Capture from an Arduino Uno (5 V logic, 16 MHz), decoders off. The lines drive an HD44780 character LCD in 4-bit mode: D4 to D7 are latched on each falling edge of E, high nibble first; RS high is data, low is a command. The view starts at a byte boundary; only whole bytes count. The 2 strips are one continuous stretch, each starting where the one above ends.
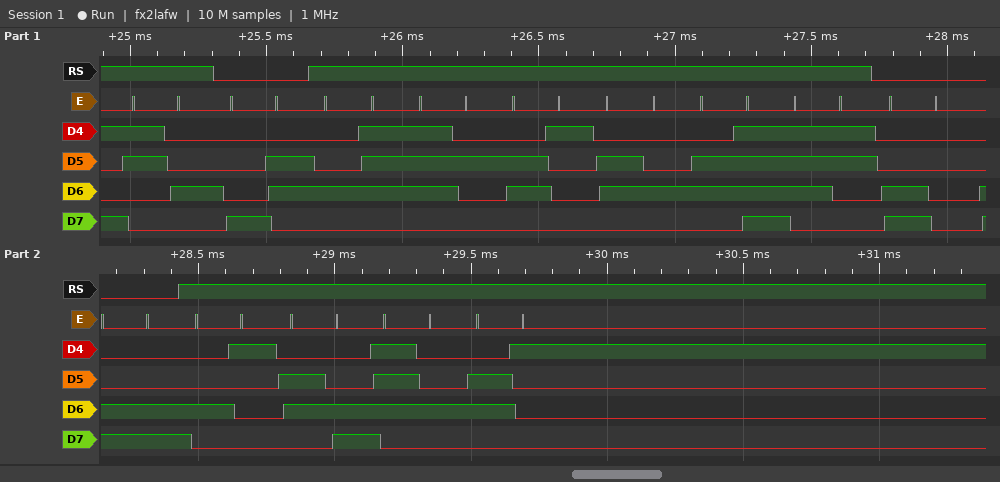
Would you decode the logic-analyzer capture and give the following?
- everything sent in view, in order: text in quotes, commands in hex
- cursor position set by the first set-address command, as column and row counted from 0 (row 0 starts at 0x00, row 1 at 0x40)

"4" 0x86 "Grados" 0xC0 0xCC "Alta"
column 6, row 0
